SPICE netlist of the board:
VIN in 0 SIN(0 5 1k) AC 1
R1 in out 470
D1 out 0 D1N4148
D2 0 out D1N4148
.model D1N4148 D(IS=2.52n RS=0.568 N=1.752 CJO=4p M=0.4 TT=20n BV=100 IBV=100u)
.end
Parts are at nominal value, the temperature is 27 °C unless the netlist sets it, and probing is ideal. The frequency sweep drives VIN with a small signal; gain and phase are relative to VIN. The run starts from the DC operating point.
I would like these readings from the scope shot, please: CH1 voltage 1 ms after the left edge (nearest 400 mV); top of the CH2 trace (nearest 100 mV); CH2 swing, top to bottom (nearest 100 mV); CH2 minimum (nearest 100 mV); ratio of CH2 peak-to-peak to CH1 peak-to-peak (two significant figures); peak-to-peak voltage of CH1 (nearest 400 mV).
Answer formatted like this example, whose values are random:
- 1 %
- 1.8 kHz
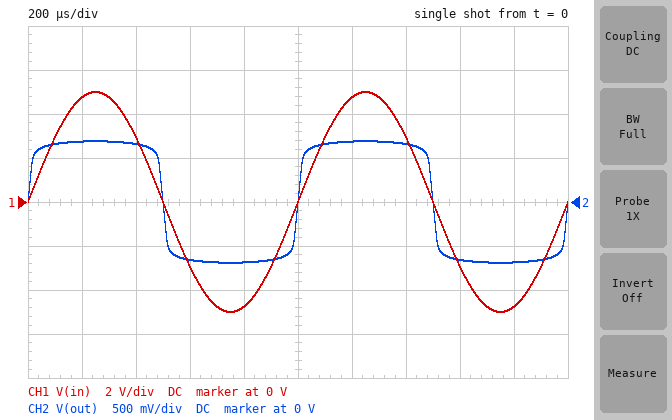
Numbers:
- 0 V
- 700 mV
- 1.4 V
- -700 mV
- 0.14
- 10.0 V
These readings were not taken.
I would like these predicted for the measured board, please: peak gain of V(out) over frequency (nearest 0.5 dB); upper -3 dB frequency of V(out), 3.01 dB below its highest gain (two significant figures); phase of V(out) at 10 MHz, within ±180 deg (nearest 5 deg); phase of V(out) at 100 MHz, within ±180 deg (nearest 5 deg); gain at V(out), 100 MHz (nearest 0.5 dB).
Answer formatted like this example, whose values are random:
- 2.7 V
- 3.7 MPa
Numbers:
- 0 dB
- 42 MHz
- -15 deg
- -65 deg
- -8.0 dB
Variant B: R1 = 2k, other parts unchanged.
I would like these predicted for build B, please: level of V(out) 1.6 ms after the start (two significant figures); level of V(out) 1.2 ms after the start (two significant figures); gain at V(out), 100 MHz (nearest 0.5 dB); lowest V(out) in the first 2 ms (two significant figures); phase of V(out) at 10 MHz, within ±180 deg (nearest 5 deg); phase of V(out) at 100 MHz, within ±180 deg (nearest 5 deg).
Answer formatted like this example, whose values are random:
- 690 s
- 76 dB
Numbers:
- -590 mV
- 620 mV
- -20.0 dB
- -620 mV
- -45 deg
- -85 deg
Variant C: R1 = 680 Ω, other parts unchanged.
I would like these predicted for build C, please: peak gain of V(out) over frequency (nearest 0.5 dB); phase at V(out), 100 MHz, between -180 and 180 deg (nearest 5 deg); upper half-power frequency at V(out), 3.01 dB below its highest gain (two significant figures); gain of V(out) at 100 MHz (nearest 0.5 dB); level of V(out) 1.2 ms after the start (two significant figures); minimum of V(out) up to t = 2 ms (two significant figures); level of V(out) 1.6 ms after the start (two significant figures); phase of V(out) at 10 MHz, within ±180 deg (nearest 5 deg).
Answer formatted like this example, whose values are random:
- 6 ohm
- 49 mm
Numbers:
- 0 dB
- -75 deg
- 29 MHz
- -11.0 dB
- 670 mV
- -670 mV
- -640 mV
- -20 deg
